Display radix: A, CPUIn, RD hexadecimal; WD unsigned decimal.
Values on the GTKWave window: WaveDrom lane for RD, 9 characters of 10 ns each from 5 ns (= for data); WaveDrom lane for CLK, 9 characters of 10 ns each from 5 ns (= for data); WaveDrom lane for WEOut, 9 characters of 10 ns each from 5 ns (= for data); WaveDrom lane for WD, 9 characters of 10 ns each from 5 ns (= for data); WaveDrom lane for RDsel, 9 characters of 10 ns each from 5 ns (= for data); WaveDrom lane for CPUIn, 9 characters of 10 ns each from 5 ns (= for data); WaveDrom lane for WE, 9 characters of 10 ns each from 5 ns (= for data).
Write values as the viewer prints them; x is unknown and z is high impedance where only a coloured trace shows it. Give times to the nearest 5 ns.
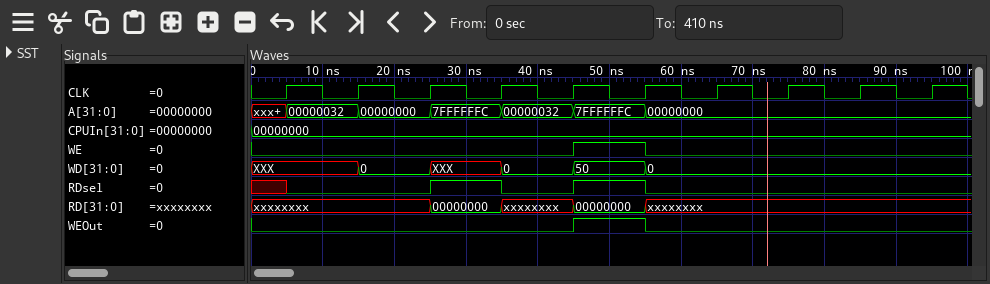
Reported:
{name: 'RD', wave: 'x.=x=x...', data: '00000000 00000000'}
{name: 'CLK', wave: 'p........'}
{name: 'WEOut', wave: '0...10...'}
{name: 'WD', wave: 'x=x===...', data: '0 0 50 0'}
{name: 'RDsel', wave: '0.1010...'}
{name: 'CPUIn', wave: '=........', data: '00000000'}
{name: 'WE', wave: '0...10...'}
